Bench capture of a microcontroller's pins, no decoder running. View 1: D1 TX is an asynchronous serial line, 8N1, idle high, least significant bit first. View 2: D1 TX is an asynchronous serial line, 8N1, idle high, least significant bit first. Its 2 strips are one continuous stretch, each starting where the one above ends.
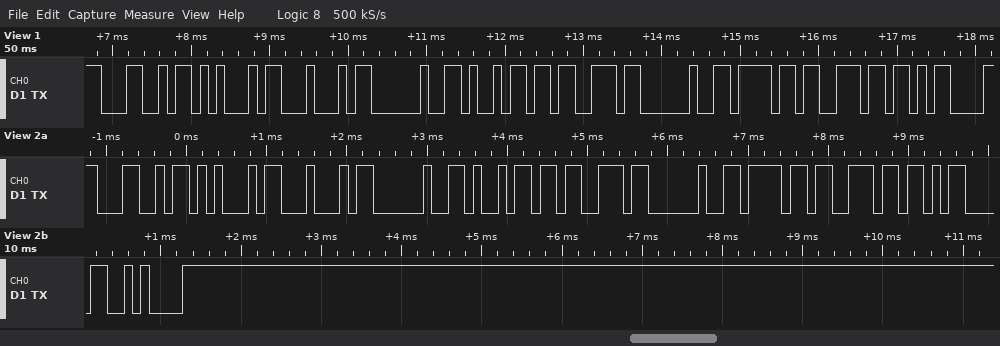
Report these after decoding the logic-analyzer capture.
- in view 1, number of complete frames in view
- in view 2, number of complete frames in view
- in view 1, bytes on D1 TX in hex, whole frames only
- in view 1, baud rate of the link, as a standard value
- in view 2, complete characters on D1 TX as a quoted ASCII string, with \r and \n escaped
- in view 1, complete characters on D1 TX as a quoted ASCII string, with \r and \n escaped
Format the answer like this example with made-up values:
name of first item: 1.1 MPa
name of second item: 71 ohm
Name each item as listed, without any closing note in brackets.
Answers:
in view 1, number of complete frames in view: 10
in view 2, number of complete frames in view: 11
in view 1, bytes on D1 TX in hex, whole frames only: 4C 45 44 20 69 73 20 6F 6E 0D
in view 1, baud rate of the link, as a standard value: 9600 baud
in view 2, complete characters on D1 TX as a quoted ASCII string, with \r and \n escaped: "LED is on\r\n"
in view 1, complete characters on D1 TX as a quoted ASCII string, with \r and \n escaped: "LED is on\r"
